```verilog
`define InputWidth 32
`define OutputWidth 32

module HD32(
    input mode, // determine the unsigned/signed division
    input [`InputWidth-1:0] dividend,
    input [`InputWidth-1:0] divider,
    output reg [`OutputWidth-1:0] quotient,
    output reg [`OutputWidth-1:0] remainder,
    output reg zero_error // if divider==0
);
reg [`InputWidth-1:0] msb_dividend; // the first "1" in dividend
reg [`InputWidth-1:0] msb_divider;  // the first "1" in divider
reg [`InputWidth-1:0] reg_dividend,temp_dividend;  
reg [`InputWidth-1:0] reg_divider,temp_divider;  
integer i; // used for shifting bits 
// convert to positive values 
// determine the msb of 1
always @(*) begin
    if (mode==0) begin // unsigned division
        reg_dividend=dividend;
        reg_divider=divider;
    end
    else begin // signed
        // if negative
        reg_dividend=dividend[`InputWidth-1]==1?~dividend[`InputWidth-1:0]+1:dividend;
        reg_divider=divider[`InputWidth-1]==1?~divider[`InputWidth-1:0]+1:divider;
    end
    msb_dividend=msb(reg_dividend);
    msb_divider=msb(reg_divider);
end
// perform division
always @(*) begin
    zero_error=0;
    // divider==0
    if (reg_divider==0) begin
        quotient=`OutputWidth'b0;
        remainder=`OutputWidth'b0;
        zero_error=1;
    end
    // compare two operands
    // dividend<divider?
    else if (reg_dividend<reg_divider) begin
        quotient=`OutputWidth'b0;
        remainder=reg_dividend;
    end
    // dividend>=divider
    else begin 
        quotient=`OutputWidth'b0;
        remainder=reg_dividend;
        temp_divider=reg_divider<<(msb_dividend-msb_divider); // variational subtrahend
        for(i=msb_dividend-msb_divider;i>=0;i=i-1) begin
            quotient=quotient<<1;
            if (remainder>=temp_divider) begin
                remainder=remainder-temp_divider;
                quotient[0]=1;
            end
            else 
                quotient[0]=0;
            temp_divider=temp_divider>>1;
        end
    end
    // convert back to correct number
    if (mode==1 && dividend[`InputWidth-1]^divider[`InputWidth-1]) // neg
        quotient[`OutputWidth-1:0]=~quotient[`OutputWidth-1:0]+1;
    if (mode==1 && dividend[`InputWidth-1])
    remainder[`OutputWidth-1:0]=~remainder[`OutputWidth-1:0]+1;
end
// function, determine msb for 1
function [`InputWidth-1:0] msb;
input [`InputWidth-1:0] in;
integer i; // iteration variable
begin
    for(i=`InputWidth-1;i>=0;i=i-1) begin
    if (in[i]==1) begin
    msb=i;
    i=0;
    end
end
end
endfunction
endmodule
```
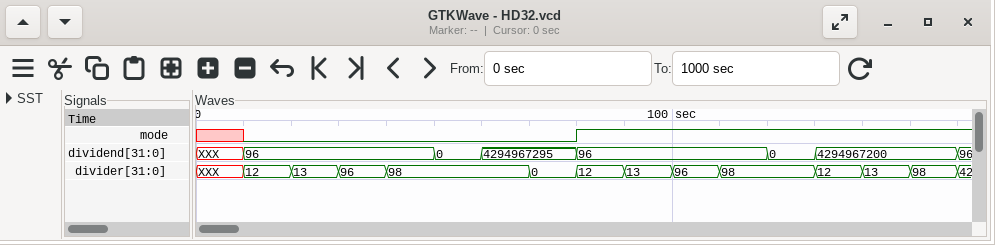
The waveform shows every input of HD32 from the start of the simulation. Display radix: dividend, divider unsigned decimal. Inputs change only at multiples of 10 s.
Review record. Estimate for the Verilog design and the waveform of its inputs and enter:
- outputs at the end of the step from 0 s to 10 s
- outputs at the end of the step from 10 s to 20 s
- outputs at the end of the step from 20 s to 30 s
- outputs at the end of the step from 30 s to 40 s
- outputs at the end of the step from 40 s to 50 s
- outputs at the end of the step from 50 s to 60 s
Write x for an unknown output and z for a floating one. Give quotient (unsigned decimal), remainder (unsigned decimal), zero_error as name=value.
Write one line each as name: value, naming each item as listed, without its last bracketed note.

outputs at the end of the step from 0 s to 10 s: quotient=x, remainder=x, zero_error=x
outputs at the end of the step from 10 s to 20 s: quotient=8, remainder=0, zero_error=0
outputs at the end of the step from 20 s to 30 s: quotient=7, remainder=5, zero_error=0
outputs at the end of the step from 30 s to 40 s: quotient=1, remainder=0, zero_error=0
outputs at the end of the step from 40 s to 50 s: quotient=0, remainder=96, zero_error=0
outputs at the end of the step from 50 s to 60 s: quotient=0, remainder=0, zero_error=0
